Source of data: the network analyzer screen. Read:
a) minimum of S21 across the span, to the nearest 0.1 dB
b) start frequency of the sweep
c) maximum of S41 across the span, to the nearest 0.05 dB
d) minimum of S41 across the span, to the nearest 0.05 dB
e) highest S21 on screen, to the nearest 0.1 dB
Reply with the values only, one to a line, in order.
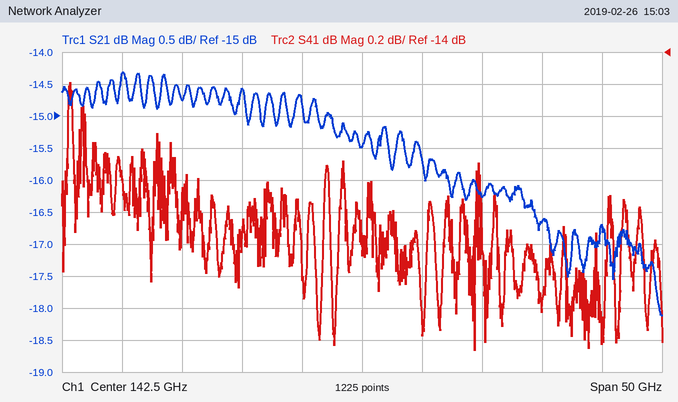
-18.1 dB
117.5 GHz
-14.20 dB
-15.85 dB
-14.3 dB
